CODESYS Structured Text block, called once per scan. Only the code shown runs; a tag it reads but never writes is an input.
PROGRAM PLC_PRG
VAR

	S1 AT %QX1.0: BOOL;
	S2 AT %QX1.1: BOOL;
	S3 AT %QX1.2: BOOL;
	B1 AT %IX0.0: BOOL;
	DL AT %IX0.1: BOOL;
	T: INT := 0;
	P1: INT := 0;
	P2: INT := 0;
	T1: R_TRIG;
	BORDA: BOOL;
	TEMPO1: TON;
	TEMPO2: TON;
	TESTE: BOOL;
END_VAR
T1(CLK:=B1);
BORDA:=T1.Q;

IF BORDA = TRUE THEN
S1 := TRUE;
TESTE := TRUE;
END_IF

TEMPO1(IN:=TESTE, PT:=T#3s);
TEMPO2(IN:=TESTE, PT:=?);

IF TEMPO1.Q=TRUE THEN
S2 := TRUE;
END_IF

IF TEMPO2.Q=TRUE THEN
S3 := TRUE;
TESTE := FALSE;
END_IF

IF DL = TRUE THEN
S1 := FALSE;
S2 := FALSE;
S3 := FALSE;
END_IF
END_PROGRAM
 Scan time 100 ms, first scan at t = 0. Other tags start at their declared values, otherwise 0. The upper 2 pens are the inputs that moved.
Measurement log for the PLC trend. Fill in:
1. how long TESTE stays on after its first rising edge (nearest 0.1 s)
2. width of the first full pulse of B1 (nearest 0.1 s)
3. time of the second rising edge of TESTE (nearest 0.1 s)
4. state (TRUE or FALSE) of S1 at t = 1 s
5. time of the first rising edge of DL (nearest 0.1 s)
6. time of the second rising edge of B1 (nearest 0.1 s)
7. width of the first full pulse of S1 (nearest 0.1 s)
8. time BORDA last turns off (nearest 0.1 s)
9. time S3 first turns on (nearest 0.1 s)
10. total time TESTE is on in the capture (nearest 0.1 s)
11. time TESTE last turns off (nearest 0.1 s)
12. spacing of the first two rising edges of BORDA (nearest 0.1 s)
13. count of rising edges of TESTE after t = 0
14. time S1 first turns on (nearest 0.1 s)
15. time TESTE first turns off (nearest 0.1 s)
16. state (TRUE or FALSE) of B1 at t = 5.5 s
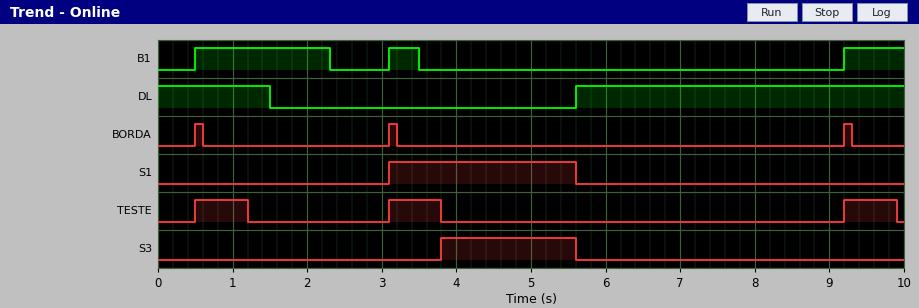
0.7 s
1.8 s
3.1 s
FALSE
5.6 s
3.1 s
2.5 s
9.3 s
3.8 s
2.1 s
9.9 s
2.6 s
3
3.1 s
1.2 s
FALSE
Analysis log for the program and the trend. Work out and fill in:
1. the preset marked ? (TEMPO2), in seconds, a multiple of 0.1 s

0.7 s
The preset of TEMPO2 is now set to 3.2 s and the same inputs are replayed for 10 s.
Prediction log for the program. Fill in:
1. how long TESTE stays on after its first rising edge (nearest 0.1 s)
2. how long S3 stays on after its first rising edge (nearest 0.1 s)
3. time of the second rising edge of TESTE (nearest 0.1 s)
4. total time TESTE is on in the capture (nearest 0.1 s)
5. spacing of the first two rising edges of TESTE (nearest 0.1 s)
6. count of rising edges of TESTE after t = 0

3.2 s
1.9 s
9.2 s
4.0 s
8.7 s
2
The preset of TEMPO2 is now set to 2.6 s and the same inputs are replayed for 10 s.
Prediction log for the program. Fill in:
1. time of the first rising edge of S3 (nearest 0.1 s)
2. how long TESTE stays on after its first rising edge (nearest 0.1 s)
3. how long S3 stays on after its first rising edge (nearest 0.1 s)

3.1 s
2.6 s
2.5 s
